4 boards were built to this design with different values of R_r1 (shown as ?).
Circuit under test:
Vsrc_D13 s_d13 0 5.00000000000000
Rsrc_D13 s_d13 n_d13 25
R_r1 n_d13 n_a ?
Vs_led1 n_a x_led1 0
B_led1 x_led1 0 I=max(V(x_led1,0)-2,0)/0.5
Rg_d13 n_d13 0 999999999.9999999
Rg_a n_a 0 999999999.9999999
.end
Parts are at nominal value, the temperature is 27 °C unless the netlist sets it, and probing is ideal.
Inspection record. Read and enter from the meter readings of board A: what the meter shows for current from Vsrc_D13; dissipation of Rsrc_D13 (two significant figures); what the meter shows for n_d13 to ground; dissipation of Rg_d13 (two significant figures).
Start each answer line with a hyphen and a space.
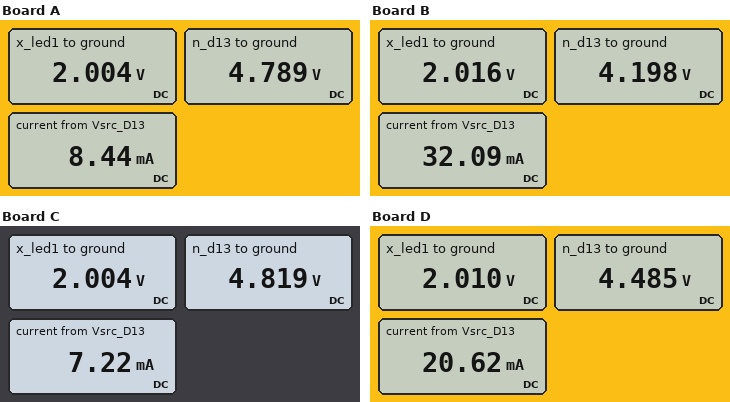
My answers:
- 8.44 mA
- 1.8 mW
- 4.789 V
- 23 nW
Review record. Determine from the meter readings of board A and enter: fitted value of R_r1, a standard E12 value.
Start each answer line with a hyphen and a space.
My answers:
- 330 Ω
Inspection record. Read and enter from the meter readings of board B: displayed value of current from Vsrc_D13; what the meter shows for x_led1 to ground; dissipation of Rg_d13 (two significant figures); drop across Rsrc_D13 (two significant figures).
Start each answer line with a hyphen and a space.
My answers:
- 32.09 mA
- 2.016 V
- 18 nW
- 800 mV
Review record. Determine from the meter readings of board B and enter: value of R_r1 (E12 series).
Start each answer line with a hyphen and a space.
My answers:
- 68 Ω
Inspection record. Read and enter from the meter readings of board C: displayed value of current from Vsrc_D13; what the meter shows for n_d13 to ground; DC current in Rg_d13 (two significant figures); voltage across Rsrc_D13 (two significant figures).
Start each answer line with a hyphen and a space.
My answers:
- 7.22 mA
- 4.819 V
- 4.8 nA
- 180 mV
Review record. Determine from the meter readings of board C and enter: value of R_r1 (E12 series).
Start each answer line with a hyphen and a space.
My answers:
- 390 Ω
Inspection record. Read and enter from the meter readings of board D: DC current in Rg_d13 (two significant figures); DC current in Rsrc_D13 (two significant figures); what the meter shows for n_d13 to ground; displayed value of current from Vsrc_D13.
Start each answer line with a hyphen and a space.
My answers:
- 4.5 nA
- 21 mA
- 4.485 V
- 20.62 mA
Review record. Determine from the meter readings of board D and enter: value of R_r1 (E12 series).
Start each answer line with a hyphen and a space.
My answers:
- 120 Ω
